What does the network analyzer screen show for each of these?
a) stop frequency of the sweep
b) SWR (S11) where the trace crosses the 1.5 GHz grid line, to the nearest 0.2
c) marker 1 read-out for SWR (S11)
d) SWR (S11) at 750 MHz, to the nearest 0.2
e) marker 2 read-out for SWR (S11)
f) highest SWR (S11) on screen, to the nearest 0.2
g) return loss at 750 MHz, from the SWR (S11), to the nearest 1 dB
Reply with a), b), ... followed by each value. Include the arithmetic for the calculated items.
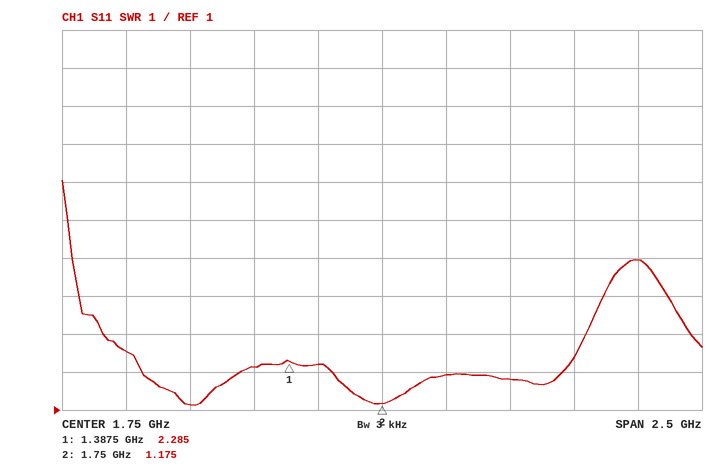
a) 3 GHz
b) 2.2
c) 2.285
d) 2.6
e) 1.175
f) 7.0
g) −20 log10((2.6 − 1)/(2.6 + 1)) ≈ 7 dB
